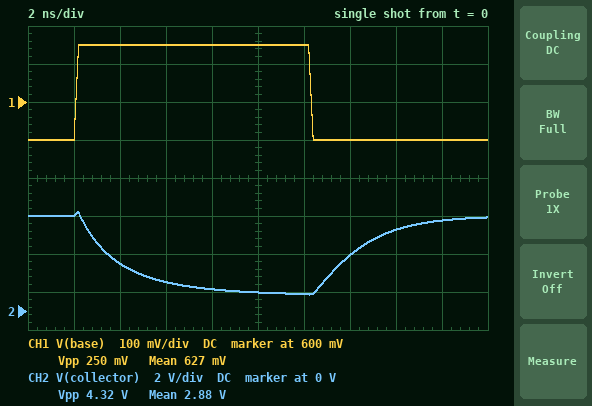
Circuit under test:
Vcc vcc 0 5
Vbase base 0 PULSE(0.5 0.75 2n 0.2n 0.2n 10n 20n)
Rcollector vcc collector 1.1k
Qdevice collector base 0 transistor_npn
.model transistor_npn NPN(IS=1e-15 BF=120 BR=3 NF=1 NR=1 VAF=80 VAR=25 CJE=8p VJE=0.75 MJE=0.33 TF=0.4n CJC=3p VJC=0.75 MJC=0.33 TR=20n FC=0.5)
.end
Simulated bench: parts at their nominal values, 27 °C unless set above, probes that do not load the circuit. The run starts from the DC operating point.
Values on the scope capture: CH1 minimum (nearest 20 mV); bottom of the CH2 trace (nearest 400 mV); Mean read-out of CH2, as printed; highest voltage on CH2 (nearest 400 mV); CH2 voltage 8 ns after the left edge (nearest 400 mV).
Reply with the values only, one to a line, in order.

500 mV
800 mV
2.88 V
5.2 V
1.2 V
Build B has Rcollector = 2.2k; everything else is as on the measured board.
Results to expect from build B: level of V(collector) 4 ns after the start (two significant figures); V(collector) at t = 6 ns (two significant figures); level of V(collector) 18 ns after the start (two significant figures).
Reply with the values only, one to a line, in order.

2.0 V
450 mV
1.9 V
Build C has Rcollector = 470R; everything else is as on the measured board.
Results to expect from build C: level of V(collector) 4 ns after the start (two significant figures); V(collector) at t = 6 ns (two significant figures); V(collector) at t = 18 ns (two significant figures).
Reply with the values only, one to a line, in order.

3.4 V
3.2 V
5.0 V
